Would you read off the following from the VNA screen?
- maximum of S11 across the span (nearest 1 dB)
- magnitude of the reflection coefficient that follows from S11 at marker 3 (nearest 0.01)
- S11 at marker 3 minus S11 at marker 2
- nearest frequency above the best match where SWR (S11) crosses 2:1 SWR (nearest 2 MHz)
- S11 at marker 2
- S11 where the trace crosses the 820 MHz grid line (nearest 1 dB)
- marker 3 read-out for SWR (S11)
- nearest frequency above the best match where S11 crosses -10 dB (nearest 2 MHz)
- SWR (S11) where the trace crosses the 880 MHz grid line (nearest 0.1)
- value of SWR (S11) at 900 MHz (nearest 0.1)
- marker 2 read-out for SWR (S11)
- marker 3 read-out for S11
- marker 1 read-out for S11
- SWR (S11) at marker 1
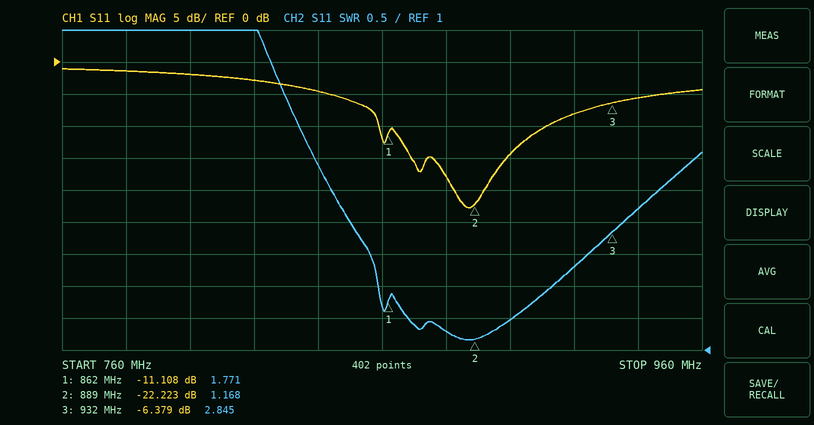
-1 dB
0.48
15.844 dB
914 MHz
-22.223 dB
-3 dB
2.845
912 MHz
1.3
1.5
1.168
-6.379 dB
-11.108 dB
1.771
